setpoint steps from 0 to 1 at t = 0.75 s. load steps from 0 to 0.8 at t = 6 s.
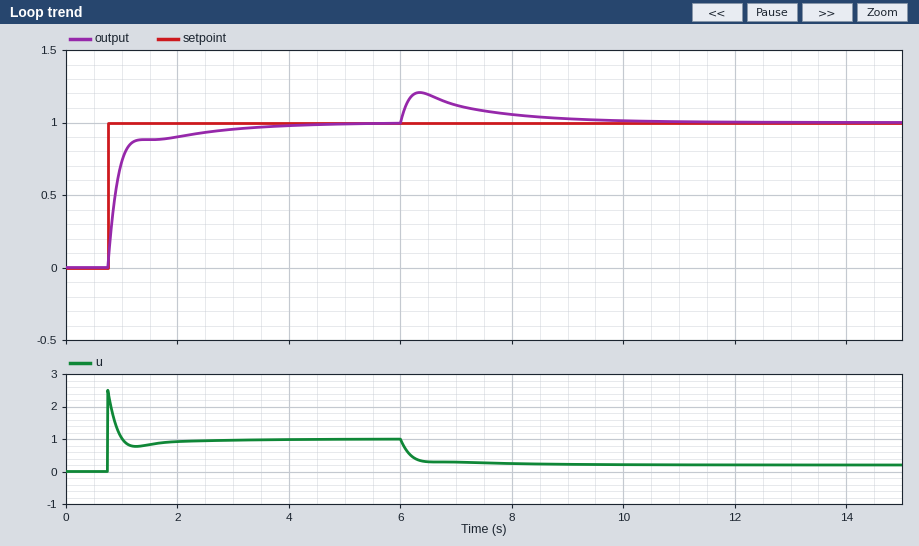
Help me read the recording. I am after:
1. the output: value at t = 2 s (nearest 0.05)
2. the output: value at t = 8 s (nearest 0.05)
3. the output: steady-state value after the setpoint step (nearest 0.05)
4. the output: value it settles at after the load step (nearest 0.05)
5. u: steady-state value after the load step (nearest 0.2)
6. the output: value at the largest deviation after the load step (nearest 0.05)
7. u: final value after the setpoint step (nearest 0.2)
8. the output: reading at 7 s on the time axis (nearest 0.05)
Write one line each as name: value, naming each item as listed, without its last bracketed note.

the output: value at t = 2 s: 0.90
the output: value at t = 8 s: 1.05
the output: steady-state value after the setpoint step: 1.00
the output: value it settles at after the load step: 1.00
u: steady-state value after the load step: 0.2
the output: value at the largest deviation after the load step: 1.20
u: final value after the setpoint step: 1.0
the output: reading at 7 s on the time axis: 1.10
